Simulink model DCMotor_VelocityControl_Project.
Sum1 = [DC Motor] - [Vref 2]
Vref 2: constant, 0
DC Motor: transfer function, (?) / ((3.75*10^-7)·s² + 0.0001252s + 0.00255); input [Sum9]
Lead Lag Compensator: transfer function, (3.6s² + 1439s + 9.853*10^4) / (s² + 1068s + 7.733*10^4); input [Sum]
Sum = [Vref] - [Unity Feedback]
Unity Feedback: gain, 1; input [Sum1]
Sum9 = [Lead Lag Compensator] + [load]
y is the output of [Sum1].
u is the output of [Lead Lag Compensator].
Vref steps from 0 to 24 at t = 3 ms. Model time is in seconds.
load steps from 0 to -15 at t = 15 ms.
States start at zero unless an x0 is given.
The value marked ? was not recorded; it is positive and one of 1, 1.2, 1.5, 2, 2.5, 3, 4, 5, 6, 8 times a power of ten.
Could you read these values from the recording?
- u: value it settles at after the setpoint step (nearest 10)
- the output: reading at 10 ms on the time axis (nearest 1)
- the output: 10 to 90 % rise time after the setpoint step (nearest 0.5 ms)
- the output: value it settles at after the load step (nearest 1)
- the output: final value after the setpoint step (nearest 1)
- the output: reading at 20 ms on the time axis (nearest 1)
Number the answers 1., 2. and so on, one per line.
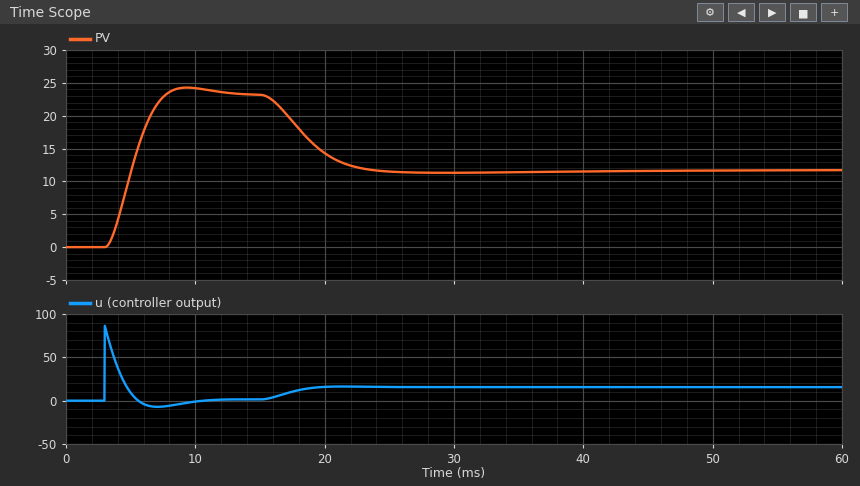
1. 0
2. 24
3. 3.0 ms
4. 12
5. 23
6. 14
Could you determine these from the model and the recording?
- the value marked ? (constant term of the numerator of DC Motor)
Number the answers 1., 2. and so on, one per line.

1. 0.05
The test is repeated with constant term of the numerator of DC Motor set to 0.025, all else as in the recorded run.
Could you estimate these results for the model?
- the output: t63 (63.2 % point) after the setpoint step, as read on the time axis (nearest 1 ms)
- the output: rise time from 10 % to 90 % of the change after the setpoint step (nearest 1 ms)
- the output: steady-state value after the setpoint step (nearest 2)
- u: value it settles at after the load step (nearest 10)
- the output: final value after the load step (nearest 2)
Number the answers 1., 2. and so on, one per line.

1. 7 ms
2. 6 ms
3. 22
4. 20
5. 12
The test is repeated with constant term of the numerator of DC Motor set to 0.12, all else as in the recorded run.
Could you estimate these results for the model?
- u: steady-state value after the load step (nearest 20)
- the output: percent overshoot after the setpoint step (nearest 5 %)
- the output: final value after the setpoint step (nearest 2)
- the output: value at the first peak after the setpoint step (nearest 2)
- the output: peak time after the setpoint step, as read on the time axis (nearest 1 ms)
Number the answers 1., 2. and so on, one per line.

1. 20
2. 20 %
3. 24
4. 28
5. 6 ms
